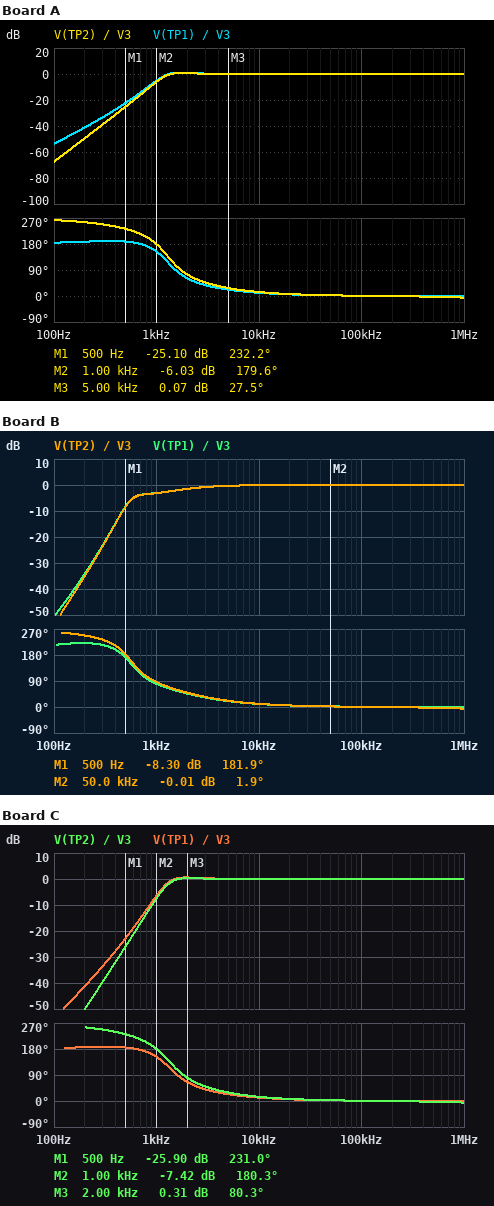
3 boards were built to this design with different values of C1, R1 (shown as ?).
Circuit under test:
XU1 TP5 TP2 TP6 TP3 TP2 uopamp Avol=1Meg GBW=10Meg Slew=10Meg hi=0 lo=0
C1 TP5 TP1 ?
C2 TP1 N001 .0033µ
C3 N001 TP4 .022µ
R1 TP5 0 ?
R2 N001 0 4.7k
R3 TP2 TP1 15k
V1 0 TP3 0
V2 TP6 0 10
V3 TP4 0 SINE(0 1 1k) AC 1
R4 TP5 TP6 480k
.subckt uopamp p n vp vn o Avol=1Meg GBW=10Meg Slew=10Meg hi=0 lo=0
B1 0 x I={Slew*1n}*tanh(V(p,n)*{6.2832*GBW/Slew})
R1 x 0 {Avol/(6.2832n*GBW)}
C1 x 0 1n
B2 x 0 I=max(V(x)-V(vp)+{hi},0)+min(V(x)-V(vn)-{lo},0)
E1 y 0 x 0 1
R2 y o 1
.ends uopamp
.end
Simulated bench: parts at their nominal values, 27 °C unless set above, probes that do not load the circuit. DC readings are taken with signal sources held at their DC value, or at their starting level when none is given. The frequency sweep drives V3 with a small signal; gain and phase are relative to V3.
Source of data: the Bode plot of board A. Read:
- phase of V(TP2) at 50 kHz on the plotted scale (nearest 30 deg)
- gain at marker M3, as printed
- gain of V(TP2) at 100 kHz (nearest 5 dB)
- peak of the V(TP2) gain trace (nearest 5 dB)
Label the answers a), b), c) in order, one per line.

a) 0 deg
b) 0.07 dB
c) 0 dB
d) 0 dB
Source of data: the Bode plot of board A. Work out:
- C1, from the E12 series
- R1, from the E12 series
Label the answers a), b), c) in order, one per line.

a) 2.2 nF
b) 220 kΩ
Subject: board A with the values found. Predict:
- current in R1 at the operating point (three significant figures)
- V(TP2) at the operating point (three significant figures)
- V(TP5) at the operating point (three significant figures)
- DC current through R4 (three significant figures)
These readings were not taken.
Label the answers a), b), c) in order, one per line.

a) 14.3 µA
b) 3.14 V
c) 3.14 V
d) 14.3 µA
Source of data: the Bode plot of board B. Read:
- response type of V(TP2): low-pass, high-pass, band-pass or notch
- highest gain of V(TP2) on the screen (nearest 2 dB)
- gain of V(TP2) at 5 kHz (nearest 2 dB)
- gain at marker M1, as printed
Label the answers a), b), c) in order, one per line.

a) high-pass
b) 0 dB
c) 0 dB
d) -8.30 dB
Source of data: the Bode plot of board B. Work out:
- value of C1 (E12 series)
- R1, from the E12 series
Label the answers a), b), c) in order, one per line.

a) 8.2 nF
b) 330 kΩ
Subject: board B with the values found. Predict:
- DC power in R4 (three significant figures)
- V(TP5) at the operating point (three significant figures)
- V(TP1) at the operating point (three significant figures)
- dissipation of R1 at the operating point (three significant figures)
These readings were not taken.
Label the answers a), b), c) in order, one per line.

a) 73.2 µW
b) 4.07 V
c) 4.07 V
d) 50.3 µW
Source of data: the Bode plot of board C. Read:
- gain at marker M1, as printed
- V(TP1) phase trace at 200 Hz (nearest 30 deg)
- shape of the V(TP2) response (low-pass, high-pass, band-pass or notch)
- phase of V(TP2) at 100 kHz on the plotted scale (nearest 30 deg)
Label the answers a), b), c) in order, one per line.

a) -25.90 dB
b) 180 deg
c) high-pass
d) 0 deg
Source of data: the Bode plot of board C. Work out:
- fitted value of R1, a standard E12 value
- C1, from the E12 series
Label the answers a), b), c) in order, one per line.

a) 150 kΩ
b) 2.7 nF
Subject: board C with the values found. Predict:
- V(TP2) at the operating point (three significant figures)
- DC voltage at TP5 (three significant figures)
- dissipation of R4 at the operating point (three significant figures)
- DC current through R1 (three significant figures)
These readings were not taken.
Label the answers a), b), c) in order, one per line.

a) 2.38 V
b) 2.38 V
c) 121 µW
d) 15.9 µA
